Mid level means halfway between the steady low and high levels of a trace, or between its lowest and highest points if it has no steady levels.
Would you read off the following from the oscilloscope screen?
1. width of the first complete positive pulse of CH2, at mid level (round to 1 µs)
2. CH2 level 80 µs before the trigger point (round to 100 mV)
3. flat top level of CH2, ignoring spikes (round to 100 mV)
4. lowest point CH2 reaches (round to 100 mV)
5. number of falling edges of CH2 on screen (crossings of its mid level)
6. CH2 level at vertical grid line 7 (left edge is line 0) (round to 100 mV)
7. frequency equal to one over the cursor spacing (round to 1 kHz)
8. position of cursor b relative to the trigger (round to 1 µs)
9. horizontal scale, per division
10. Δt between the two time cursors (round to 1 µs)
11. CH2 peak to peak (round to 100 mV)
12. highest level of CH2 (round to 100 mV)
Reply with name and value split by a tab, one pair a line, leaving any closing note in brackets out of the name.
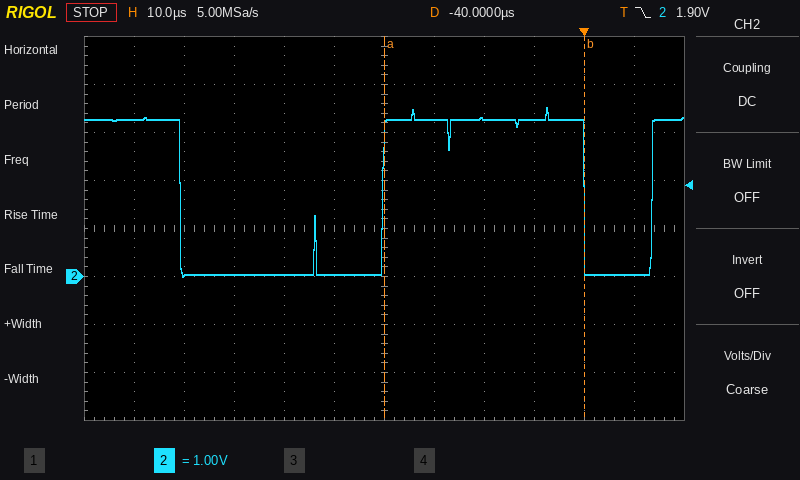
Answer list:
width of the first complete positive pulse of CH2, at mid level	40 µs
CH2 level 80 µs before the trigger point	100 mV
flat top level of CH2, ignoring spikes	3.3 V
lowest point CH2 reaches	0.0 V
number of falling edges of CH2 on screen	2
CH2 level at vertical grid line 7 (left edge is line 0)	3.3 V
frequency equal to one over the cursor spacing	25 kHz
position of cursor b relative to the trigger	0 µs
horizontal scale, per division	10 µs
Δt between the two time cursors	40 µs
CH2 peak to peak	3.5 V
highest level of CH2	3.5 V
